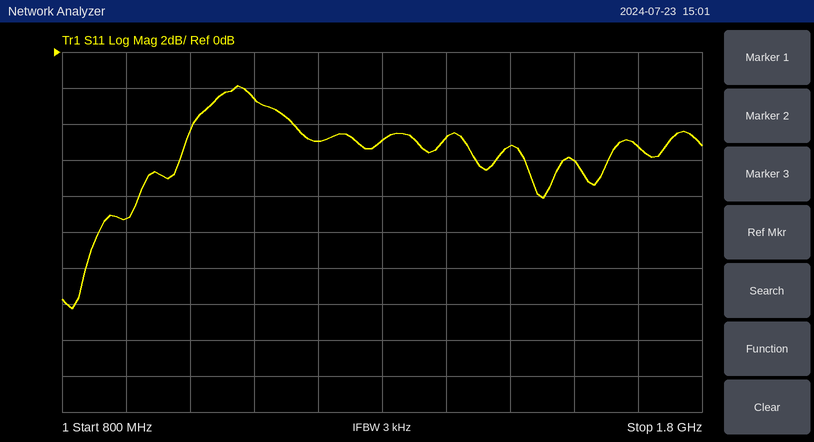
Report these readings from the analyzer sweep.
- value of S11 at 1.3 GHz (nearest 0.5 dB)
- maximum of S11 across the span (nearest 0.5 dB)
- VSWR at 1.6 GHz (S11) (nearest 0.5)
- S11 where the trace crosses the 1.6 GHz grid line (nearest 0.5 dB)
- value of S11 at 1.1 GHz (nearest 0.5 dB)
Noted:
-5.0 dB
-2.0 dB
3.0
-6.0 dB
-2.5 dB
